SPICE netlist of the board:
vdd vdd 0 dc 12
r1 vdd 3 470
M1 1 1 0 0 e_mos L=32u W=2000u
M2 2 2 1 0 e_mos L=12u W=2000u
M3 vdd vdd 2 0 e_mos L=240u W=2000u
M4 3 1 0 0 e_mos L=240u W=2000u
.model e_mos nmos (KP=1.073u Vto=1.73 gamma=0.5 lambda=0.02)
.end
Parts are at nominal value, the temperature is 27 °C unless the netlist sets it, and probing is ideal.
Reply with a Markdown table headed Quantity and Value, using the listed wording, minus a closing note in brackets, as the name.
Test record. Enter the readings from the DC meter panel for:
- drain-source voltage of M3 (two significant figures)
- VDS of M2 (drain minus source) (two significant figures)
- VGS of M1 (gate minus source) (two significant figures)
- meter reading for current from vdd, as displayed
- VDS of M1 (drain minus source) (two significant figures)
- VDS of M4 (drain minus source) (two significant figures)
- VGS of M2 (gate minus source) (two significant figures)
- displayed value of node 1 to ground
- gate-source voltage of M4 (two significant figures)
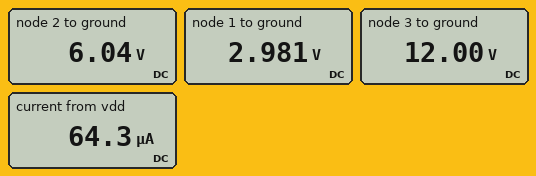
| Quantity | Value |
|---|---|
| drain-source voltage of M3 | 6.0 V |
| VDS of M2 (drain minus source) | 3.1 V |
| VGS of M1 (gate minus source) | 3.0 V |
| meter reading for current from vdd, as displayed | 64.3 µA |
| VDS of M1 (drain minus source) | 3.0 V |
| VDS of M4 (drain minus source) | 12 V |
| VGS of M2 (gate minus source) | 3.1 V |
| displayed value of node 1 to ground | 2.981 V |
| gate-source voltage of M4 | 3.0 V |
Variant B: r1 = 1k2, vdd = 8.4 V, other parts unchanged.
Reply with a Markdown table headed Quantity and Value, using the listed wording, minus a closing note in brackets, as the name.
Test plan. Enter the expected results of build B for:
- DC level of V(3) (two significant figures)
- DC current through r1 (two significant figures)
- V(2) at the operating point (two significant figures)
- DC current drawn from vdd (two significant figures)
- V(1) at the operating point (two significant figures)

| Quantity | Value |
|---|---|
| DC level of V(3) | 8.4 V |
| DC current through r1 | 1.1 µA |
| V(2) at the operating point | 4.7 V |
| DC current drawn from vdd | 8.7 µA |
| V(1) at the operating point | 2.2 V |
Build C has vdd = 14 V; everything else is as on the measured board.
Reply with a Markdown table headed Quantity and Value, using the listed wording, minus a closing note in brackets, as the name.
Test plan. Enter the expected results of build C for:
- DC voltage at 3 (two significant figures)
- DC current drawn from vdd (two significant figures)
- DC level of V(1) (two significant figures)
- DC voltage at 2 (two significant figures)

| Quantity | Value |
|---|---|
| DC voltage at 3 | 14 V |
| DC current drawn from vdd | 120 µA |
| DC level of V(1) | 3.4 V |
| DC voltage at 2 | 6.8 V |
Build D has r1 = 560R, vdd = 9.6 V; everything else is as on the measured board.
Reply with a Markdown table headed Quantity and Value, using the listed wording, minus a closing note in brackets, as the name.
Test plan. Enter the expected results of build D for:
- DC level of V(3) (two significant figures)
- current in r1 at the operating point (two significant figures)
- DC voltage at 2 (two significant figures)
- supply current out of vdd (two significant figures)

| Quantity | Value |
|---|---|
| DC level of V(3) | 9.6 V |
| current in r1 at the operating point | 2.8 µA |
| DC voltage at 2 | 5.1 V |
| supply current out of vdd | 21 µA |
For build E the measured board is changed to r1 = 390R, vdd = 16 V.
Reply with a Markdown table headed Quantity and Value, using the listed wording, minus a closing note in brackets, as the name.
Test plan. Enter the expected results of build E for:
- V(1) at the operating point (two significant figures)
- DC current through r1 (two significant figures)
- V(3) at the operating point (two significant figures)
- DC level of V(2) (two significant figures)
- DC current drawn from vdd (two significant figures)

| Quantity | Value |
|---|---|
| V(1) at the operating point | 3.9 V |
| DC current through r1 | 27 µA |
| V(3) at the operating point | 16 V |
| DC level of V(2) | 7.6 V |
| DC current drawn from vdd | 190 µA |
